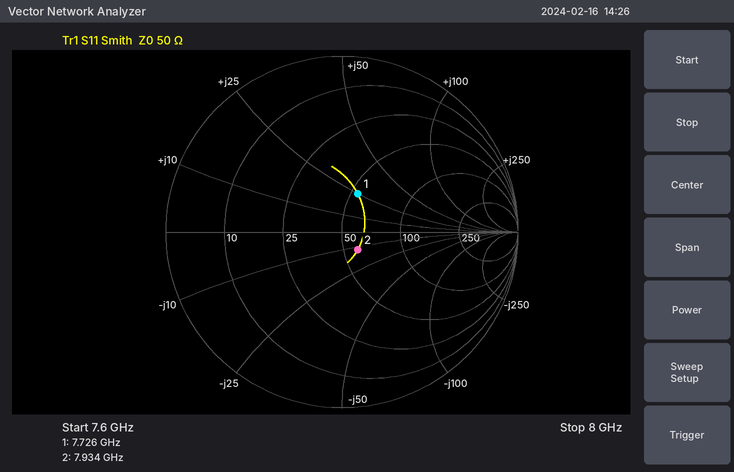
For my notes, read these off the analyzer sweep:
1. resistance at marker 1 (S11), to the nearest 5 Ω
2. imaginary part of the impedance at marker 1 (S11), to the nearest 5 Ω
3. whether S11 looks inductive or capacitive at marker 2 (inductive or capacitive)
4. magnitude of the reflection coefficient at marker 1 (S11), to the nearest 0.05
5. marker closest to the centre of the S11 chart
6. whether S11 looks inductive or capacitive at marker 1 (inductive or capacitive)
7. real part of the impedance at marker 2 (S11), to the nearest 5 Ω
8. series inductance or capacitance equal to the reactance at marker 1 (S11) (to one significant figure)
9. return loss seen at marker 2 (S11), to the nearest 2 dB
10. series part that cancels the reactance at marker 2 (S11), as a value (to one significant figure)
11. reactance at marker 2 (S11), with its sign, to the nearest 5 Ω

55 Ω
+25 Ω
capacitive
0.25
marker 2
inductive
60 Ω
500 pH
18 dB
200 pH
-10 Ω
